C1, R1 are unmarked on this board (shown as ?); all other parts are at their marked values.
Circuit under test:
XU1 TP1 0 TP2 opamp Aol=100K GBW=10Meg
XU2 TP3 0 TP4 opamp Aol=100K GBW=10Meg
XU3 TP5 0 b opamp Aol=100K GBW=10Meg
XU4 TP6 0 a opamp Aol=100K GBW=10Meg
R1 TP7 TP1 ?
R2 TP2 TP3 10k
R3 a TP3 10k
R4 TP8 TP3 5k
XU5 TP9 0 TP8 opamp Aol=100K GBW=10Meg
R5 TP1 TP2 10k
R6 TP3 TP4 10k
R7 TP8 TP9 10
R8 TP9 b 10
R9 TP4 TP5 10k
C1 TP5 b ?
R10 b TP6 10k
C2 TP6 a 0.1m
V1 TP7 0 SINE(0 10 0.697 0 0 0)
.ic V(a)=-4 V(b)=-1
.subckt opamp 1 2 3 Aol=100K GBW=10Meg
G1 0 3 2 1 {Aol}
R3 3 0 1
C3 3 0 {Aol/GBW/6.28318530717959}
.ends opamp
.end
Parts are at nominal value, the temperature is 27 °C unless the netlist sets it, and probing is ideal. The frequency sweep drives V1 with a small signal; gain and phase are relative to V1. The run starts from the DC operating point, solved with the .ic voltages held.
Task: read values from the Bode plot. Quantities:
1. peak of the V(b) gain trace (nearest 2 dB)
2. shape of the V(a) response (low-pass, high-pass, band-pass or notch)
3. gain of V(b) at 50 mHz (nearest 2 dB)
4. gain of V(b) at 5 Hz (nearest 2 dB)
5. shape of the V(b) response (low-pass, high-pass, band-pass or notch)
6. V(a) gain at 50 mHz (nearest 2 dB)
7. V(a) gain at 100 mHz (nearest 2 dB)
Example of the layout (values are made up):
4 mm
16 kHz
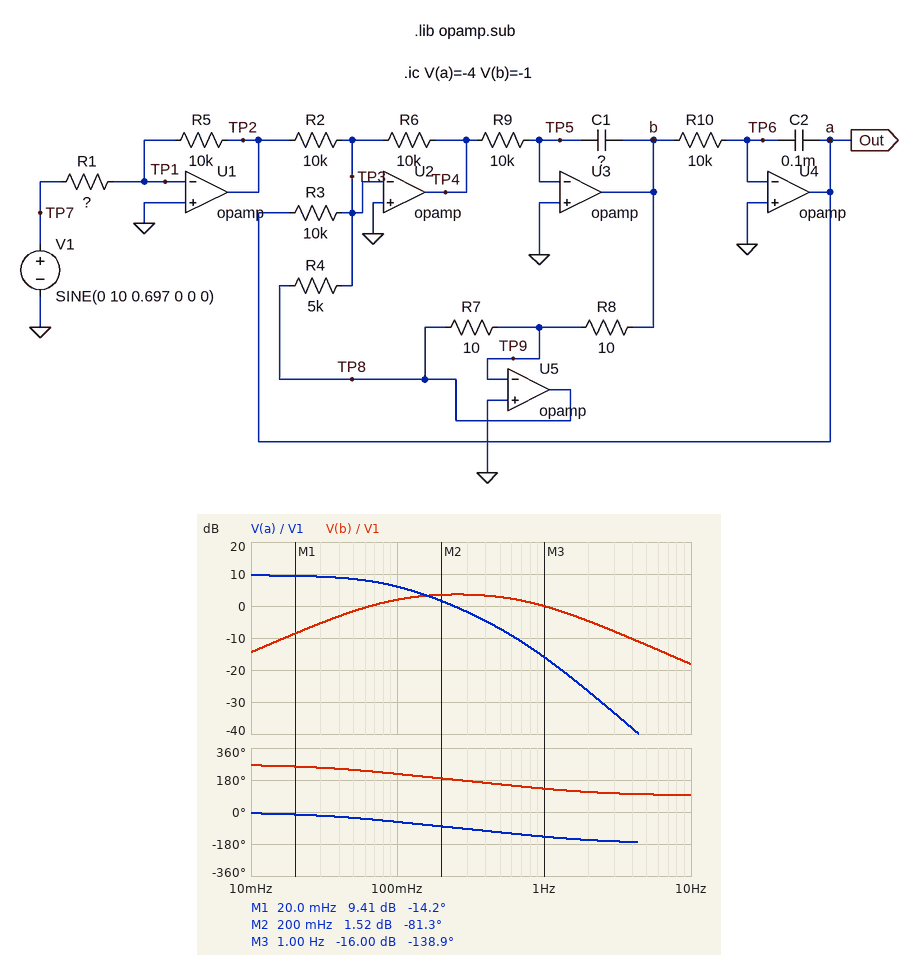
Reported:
4 dB
low-pass
-2 dB
-12 dB
band-pass
8 dB
6 dB
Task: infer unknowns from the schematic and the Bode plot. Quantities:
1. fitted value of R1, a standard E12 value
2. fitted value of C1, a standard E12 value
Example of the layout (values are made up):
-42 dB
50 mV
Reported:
3.3 kΩ
39 µF
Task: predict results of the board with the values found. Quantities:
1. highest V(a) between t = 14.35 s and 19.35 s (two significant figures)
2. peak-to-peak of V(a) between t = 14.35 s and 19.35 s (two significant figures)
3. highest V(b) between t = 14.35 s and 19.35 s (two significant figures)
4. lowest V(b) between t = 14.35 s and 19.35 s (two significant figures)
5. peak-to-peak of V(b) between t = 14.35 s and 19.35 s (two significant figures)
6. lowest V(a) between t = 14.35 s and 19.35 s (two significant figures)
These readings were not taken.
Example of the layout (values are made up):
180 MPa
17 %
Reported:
2.8 V
5.6 V
12 V
-12 V
24 V
-2.8 V
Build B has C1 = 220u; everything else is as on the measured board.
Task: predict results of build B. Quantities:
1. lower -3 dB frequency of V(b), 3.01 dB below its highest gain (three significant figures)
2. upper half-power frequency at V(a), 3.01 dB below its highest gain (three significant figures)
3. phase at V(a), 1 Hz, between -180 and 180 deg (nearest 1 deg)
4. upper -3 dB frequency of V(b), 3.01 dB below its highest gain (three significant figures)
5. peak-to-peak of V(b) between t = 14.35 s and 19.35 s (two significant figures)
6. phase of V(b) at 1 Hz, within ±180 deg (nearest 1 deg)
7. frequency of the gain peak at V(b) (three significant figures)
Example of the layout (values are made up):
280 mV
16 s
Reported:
57.1 mHz
112 mHz
-172 deg
202 mHz
6.3 V
98 deg
107 mHz
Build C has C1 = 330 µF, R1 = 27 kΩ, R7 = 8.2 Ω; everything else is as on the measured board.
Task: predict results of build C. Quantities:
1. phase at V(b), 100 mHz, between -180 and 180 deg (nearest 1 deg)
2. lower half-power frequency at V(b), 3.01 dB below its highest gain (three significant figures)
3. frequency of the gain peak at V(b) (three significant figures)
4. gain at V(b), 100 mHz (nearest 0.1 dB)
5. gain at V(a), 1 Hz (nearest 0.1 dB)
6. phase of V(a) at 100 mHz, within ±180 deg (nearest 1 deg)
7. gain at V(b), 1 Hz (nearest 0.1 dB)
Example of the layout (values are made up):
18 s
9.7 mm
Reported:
164 deg
56.6 mHz
87.6 mHz
-13.3 dB
-50.9 dB
-106 deg
-34.9 dB
